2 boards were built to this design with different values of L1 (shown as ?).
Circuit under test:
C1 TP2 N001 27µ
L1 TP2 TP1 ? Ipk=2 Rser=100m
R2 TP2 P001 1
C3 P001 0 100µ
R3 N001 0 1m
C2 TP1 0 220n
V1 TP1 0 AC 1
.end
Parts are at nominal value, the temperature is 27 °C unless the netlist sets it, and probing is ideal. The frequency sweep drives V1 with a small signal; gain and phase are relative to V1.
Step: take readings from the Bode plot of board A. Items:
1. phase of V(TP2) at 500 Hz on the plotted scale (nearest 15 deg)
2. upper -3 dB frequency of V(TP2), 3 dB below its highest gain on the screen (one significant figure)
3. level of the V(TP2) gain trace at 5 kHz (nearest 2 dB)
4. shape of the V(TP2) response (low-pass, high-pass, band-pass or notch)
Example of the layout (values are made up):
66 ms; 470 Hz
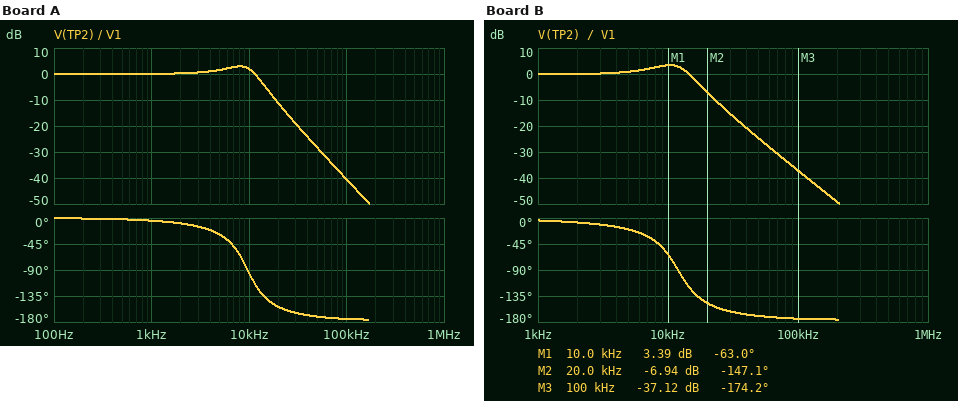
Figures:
0 deg; 10 kHz; 2 dB; low-pass
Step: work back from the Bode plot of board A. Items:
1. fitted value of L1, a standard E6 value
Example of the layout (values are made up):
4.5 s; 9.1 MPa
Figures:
10 µH
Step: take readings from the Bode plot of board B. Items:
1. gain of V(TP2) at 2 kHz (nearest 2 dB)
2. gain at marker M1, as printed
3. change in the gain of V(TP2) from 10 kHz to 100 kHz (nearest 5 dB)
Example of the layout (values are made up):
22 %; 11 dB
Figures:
0 dB; 3.39 dB; -40 dB
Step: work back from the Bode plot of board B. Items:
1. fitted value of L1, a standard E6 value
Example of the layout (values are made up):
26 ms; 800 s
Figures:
6.8 µH
